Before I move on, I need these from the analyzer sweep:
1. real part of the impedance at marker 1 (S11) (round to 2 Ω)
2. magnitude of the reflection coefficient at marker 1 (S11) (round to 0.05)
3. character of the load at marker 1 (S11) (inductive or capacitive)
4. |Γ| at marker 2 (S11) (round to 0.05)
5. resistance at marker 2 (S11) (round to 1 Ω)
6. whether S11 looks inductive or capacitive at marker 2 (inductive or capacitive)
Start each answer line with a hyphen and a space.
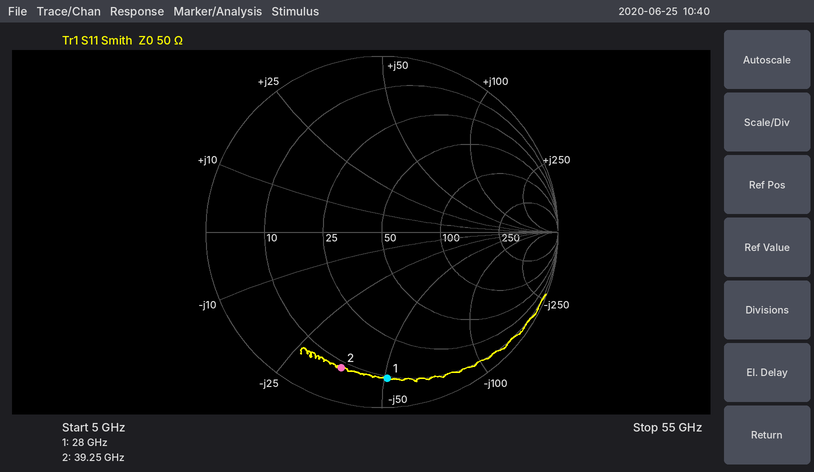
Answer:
- 10 Ω
- 0.85
- capacitive
- 0.80
- 8 Ω
- capacitive
